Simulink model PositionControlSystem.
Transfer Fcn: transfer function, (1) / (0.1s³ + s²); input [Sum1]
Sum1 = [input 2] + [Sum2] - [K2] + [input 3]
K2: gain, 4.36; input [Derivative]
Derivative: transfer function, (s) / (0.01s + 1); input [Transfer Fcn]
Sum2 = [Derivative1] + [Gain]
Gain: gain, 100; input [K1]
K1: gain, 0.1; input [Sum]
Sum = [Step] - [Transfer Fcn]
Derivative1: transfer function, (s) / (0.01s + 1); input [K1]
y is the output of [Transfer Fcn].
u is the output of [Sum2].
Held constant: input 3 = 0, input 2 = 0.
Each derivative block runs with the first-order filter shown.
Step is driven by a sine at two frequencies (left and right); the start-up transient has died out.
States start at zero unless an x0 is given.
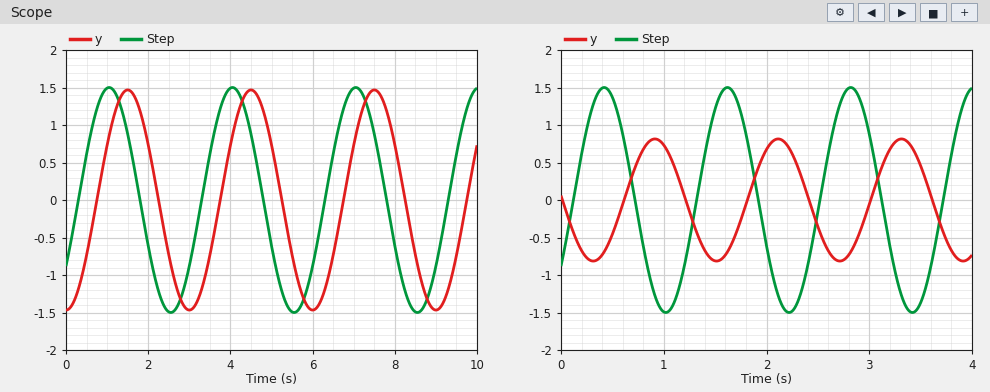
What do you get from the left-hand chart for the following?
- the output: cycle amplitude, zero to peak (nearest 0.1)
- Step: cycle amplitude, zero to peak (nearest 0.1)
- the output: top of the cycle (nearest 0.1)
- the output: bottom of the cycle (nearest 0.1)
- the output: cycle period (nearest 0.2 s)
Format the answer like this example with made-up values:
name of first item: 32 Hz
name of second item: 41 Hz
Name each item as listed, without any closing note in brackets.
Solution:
the output: cycle amplitude, zero to peak: 1.5
Step: cycle amplitude, zero to peak: 1.5
the output: top of the cycle: 1.5
the output: bottom of the cycle: -1.5
the output: cycle period: 3.0 s
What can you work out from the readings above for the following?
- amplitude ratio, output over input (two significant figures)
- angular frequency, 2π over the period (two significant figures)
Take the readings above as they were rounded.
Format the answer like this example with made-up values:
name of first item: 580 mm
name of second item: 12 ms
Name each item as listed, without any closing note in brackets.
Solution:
amplitude ratio, output over input: 1.0
angular frequency, 2π over the period: 2.1 rad/s
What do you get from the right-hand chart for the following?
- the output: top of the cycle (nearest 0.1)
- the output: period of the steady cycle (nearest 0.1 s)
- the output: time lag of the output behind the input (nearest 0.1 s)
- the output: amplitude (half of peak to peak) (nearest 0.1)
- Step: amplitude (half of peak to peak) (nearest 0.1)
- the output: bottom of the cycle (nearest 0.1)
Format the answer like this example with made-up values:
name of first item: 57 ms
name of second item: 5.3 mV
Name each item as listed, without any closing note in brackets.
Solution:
the output: top of the cycle: 0.8
the output: period of the steady cycle: 1.2 s
the output: time lag of the output behind the input: 0.5 s
the output: amplitude (half of peak to peak): 0.8
Step: amplitude (half of peak to peak): 1.5
the output: bottom of the cycle: -0.8
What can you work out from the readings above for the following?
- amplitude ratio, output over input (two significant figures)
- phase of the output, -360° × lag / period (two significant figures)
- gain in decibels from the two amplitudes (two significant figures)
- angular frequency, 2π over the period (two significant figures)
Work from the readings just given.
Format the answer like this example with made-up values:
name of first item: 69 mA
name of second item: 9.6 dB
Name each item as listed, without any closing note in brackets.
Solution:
amplitude ratio, output over input: 0.53
phase of the output, -360° × lag / period: -150°
gain in decibels from the two amplitudes: -5.5 dB
angular frequency, 2π over the period: 5.2 rad/s
